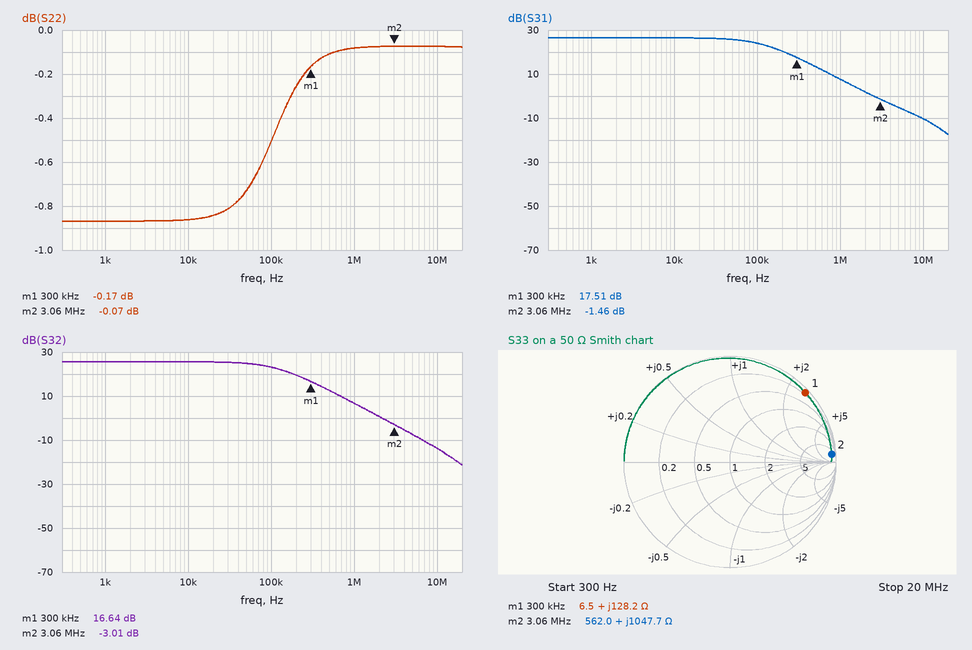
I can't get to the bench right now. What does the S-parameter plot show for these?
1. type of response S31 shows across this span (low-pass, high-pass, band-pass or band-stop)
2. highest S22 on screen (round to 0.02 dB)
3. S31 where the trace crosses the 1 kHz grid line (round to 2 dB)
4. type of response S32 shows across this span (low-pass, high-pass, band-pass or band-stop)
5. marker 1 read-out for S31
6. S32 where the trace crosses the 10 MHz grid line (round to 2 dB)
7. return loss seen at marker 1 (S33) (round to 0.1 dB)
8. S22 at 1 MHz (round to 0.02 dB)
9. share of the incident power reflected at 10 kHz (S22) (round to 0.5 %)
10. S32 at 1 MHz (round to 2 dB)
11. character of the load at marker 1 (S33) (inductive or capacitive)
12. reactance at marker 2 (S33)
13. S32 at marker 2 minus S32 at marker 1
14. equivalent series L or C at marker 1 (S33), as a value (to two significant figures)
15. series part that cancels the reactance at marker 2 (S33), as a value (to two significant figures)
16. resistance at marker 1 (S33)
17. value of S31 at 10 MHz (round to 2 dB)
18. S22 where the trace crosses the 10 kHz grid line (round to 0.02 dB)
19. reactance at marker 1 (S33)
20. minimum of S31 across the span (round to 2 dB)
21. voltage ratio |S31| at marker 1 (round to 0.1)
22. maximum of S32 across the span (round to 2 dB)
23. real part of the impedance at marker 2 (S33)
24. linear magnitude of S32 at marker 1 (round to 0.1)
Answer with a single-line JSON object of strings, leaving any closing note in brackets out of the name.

{"type of response S31 shows across this span": "low-pass", "highest S22 on screen": "-0.08 dB", "S31 where the trace crosses the 1 kHz grid line": "26 dB", "type of response S32 shows across this span": "low-pass", "marker 1 read-out for S31": "17.51 dB", "S32 where the trace crosses the 10 MHz grid line": "-14 dB", "return loss seen at marker 1 (S33)": "0.3 dB", "S22 at 1 MHz": "-0.08 dB", "share of the incident power reflected at 10 kHz (S22)": "82.0 %", "S32 at 1 MHz": "6 dB", "character of the load at marker 1 (S33)": "inductive", "reactance at marker 2": "+1047.7 Ω", "S32 at marker 2 minus S32 at marker 1": "-19.65 dB", "equivalent series L or C at marker 1 (S33), as a value": "68 µH", "series part that cancels the reactance at marker 2 (S33), as a value": "50 pF", "resistance at marker 1": "6.5 Ω", "value of S31 at 10 MHz": "-10 dB", "S22 where the trace crosses the 10 kHz grid line": "-0.86 dB", "reactance at marker 1": "+128.2 Ω", "minimum of S31 across the span": "-18 dB", "voltage ratio |S31| at marker 1": "7.5", "maximum of S32 across the span": "26 dB", "real part of the impedance at marker 2": "562.0 Ω", "linear magnitude of S32 at marker 1": "6.8"}
